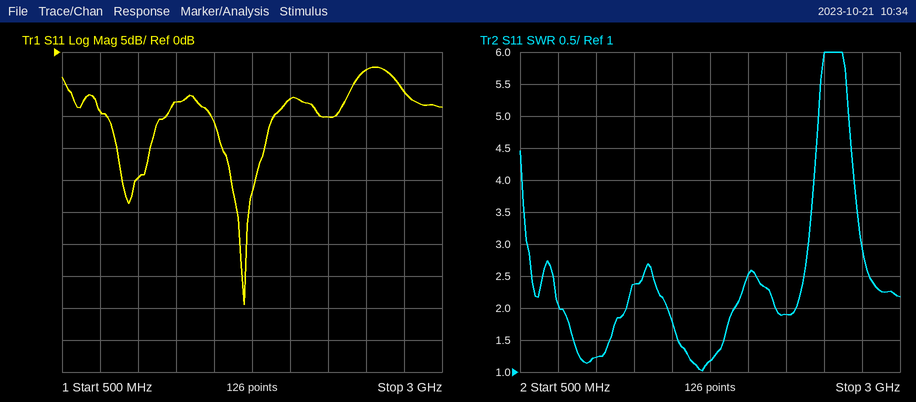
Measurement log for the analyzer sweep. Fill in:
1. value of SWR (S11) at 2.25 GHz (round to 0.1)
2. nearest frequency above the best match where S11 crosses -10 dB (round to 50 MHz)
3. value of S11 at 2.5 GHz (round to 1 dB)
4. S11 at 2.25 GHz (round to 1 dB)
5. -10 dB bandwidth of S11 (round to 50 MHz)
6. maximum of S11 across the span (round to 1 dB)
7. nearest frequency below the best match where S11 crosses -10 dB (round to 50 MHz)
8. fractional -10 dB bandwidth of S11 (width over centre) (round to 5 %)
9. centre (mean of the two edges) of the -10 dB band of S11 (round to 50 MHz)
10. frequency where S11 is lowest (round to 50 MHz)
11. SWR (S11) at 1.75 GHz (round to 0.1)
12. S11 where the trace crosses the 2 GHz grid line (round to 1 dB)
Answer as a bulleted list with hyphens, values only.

- 1.9
- 1.90 GHz
- -3 dB
- -10 dB
- 400 MHz
- -2 dB
- 1.50 GHz
- 25 %
- 1.70 GHz
- 1.70 GHz
- 1.2
- -7 dB
